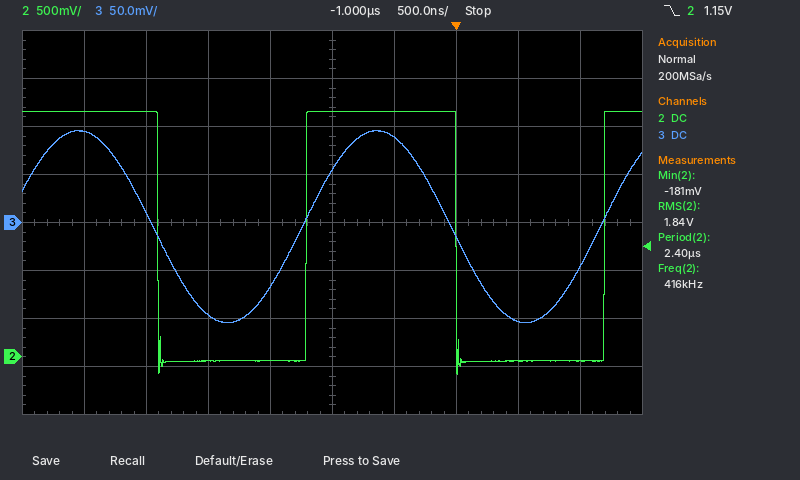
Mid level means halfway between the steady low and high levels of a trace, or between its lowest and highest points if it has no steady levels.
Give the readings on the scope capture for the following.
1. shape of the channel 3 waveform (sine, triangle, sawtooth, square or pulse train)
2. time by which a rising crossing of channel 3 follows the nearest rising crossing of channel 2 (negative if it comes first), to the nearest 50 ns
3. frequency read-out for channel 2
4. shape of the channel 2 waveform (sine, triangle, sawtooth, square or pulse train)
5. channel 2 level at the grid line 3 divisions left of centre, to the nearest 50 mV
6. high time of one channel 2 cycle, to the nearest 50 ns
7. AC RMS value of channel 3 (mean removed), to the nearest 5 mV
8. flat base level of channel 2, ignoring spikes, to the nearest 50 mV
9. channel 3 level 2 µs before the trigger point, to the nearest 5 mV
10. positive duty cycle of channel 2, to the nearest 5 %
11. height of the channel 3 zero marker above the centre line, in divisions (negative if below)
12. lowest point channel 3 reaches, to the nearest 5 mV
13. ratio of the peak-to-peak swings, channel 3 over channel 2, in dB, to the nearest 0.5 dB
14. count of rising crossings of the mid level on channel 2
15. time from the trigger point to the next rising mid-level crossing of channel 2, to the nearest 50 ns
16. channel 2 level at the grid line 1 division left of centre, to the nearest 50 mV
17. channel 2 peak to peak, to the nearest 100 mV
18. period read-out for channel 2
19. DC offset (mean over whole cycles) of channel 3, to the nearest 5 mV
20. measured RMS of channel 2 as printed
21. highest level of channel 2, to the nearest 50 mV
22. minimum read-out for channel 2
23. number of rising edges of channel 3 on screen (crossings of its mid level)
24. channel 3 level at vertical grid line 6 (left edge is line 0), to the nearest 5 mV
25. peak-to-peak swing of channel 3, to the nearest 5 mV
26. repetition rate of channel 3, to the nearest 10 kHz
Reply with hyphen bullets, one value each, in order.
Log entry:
- sine
- -50 ns
- 416 kHz
- square
- 2.55 V
- 1.20 µs
- 70 mV
- -50 mV
- -95 mV
- 50 %
- 0.0 div
- -105 mV
- -22.5 dB
- 2
- 1.20 µs
- -50 mV
- 2.70 V
- 2.40 µs
- -5 mV
- 1.84 V
- 2.55 V
- -181 mV
- 2
- 90 mV
- 200 mV
- 420 kHz
